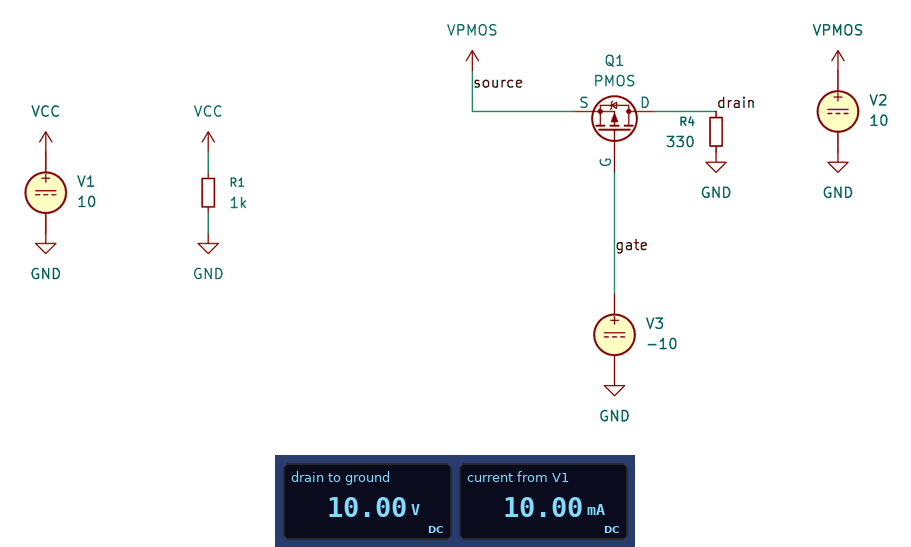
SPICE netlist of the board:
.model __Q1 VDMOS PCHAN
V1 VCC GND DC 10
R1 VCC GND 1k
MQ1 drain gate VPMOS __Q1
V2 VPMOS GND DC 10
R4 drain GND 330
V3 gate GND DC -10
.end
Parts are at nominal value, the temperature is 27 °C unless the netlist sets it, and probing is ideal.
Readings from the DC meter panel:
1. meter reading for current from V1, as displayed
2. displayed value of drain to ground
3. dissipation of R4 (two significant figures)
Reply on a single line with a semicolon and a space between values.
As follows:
10.00 mA; 10.00 V; 300 mW
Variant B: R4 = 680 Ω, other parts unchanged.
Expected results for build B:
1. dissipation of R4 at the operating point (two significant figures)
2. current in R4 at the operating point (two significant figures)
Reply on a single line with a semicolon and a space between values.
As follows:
150 mW; 15 mA
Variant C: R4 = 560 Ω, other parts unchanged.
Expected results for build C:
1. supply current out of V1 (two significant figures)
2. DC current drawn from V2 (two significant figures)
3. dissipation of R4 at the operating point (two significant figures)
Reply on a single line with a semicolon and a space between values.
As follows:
10 mA; 18 mA; 180 mW
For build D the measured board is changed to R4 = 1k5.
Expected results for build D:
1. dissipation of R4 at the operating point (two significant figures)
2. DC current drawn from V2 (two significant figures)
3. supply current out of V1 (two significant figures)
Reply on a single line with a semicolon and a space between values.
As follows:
67 mW; 6.7 mA; 10 mA
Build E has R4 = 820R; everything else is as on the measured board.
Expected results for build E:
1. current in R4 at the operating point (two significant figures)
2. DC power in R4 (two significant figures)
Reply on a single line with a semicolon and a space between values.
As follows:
12 mA; 120 mW
